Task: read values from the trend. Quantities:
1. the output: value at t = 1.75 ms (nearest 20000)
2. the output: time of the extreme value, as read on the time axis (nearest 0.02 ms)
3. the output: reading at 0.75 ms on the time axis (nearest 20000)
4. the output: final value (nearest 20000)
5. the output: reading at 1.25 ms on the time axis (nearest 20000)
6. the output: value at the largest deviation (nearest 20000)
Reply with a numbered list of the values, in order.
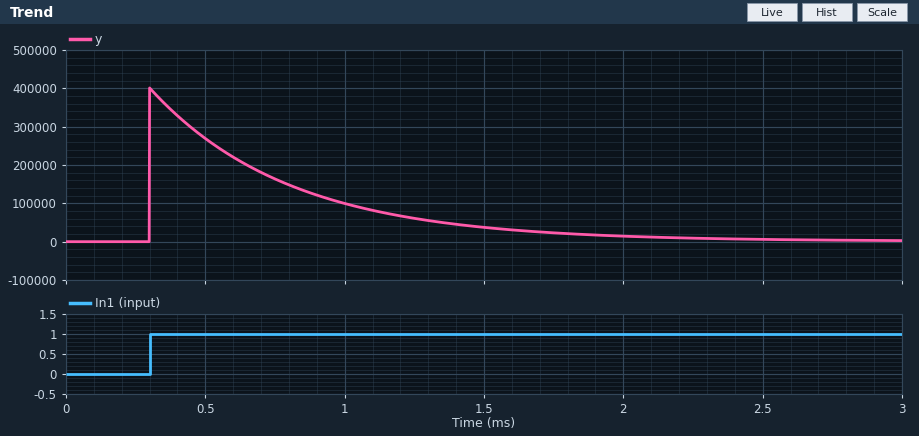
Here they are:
1. 20000
2. 0.30 ms
3. 160000
4. 0
5. 60000
6. 400000
